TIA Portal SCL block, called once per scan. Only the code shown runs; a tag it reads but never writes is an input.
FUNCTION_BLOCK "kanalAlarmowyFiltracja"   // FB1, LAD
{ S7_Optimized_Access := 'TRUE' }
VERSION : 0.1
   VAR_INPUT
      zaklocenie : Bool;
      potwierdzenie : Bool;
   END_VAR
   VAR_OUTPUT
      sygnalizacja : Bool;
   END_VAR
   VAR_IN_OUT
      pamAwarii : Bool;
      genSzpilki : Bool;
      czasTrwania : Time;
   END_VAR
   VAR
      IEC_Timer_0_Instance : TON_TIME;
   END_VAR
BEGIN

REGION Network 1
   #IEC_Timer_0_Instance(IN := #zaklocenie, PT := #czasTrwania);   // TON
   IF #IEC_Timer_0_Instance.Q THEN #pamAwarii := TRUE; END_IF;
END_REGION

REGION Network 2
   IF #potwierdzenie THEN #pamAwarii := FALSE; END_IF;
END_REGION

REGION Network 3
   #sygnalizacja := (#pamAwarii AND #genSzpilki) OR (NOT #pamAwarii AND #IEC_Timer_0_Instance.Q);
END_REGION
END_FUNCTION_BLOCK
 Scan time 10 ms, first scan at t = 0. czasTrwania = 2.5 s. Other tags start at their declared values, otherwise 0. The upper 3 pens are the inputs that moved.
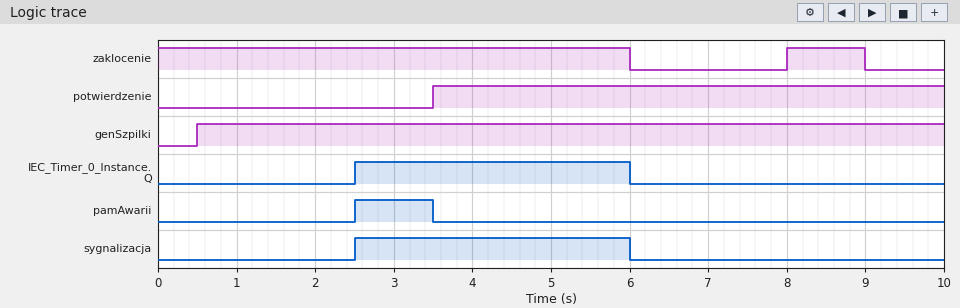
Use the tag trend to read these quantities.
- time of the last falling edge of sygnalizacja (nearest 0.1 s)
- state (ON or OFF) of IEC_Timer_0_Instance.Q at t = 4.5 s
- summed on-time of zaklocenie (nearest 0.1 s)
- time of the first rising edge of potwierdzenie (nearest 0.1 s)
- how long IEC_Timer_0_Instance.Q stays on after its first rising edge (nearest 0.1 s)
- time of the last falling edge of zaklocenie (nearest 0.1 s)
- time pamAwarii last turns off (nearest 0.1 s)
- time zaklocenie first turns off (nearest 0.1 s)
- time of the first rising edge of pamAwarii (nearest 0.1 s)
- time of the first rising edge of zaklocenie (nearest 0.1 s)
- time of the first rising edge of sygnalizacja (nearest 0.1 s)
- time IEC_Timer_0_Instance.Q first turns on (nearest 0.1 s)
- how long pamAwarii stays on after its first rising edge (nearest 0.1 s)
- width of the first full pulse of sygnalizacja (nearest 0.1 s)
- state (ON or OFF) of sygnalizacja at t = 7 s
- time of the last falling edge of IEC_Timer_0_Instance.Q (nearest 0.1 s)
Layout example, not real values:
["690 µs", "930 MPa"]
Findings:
["6.0 s", "ON", "7.0 s", "3.5 s", "3.5 s", "9.0 s", "3.5 s", "6.0 s", "2.5 s", "8.0 s", "2.5 s", "2.5 s", "1.0 s", "3.5 s", "OFF", "6.0 s"]
